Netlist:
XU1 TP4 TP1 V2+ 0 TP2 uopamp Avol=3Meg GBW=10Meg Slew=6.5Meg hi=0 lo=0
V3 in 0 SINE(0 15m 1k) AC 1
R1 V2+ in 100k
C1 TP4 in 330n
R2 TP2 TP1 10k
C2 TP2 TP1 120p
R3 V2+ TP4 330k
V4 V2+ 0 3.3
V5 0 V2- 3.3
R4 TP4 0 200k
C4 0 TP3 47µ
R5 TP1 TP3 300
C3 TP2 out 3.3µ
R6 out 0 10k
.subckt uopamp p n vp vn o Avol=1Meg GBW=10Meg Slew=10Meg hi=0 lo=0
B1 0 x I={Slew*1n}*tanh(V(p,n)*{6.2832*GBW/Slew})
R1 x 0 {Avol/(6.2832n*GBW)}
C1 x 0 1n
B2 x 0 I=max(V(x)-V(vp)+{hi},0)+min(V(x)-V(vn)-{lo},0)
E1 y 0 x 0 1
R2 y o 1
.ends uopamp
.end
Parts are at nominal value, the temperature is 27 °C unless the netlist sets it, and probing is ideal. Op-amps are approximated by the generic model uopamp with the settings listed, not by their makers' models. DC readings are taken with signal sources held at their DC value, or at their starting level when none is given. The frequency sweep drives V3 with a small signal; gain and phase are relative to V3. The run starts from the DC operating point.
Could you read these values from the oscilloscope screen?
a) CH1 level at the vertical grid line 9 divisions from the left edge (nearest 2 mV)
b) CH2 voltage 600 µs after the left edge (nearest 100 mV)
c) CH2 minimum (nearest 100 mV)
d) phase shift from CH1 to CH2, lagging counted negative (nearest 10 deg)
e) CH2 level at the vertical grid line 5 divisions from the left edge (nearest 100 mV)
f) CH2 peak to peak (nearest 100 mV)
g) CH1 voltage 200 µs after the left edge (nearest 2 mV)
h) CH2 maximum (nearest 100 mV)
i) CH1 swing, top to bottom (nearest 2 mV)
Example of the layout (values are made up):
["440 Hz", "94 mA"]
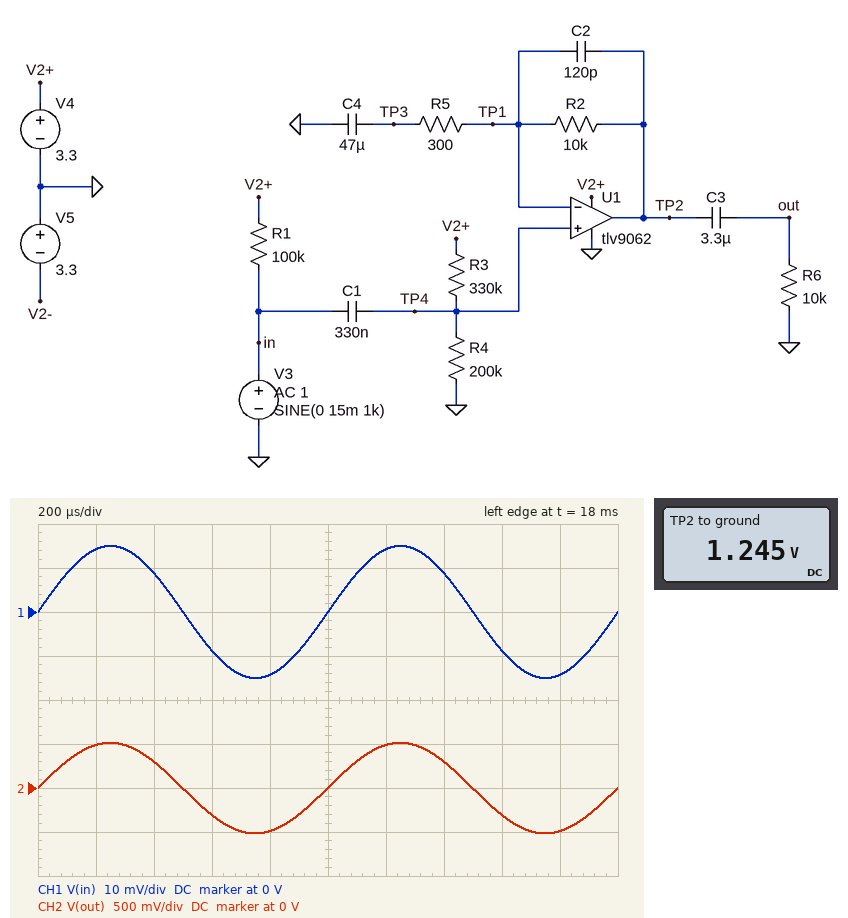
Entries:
["-14 mV", "-300 mV", "-500 mV", "0 deg", "0 V", "1.0 V", "14 mV", "500 mV", "30 mV"]
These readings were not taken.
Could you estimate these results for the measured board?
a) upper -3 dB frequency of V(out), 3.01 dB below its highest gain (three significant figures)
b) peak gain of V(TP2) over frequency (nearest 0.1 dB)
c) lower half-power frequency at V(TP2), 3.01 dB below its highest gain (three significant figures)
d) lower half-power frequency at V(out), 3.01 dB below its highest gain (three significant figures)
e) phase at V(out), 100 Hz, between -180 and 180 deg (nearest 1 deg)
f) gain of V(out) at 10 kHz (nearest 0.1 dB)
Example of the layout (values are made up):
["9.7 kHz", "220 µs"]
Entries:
["91.8 kHz", "30.7 dB", "12.4 Hz", "13.9 Hz", "11 deg", "30.7 dB"]
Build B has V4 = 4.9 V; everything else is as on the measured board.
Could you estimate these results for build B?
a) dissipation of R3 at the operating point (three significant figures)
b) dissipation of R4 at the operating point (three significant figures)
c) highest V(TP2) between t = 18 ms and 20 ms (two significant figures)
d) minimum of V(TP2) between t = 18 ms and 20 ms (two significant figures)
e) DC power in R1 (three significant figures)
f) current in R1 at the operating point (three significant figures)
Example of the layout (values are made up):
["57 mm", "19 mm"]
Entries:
["28.2 µW", "17.1 µW", "2.4 V", "1.3 V", "240 µW", "49.0 µA"]
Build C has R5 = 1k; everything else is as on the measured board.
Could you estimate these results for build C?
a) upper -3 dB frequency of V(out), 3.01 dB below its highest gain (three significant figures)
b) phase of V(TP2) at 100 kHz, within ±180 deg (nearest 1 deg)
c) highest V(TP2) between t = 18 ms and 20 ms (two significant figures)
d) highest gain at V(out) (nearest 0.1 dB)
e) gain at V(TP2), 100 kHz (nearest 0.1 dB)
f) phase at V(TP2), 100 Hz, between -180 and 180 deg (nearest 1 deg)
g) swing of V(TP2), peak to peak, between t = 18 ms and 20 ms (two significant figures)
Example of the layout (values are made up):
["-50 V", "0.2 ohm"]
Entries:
["118 kHz", "-37 deg", "1.4 V", "20.8 dB", "18.5 dB", "4 deg", "330 mV"]
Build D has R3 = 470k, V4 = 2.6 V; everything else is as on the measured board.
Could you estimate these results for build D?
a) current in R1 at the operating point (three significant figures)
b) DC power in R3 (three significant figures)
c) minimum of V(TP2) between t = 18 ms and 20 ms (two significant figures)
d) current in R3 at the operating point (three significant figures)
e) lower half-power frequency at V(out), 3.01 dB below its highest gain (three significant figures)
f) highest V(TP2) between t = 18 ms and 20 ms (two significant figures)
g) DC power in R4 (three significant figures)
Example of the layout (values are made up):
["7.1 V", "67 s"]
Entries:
["26.0 µA", "7.08 µW", "260 mV", "3.88 µA", "13.7 Hz", "1.3 V", "3.01 µW"]
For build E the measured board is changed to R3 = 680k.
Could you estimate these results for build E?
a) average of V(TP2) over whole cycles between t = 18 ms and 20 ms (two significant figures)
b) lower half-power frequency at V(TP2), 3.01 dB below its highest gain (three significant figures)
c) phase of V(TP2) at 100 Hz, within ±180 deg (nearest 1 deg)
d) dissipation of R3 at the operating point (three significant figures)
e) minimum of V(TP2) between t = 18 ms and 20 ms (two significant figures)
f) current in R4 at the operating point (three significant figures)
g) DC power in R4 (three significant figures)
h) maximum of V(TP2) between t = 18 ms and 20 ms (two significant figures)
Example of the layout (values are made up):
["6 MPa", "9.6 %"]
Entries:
["750 mV", "12.1 Hz", "8 deg", "9.56 µW", "230 mV", "3.75 µA", "2.81 µW", "1.3 V"]
